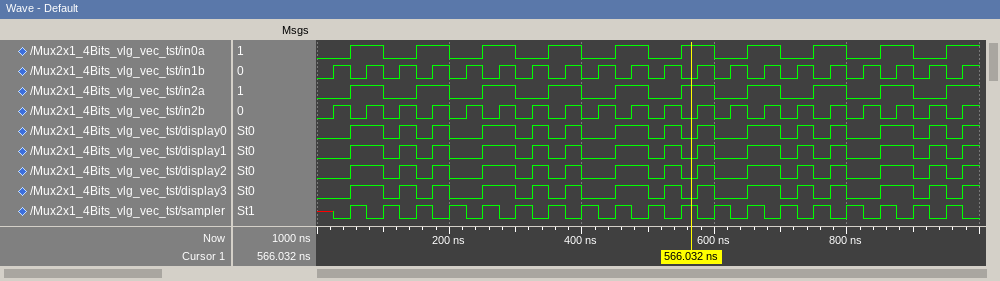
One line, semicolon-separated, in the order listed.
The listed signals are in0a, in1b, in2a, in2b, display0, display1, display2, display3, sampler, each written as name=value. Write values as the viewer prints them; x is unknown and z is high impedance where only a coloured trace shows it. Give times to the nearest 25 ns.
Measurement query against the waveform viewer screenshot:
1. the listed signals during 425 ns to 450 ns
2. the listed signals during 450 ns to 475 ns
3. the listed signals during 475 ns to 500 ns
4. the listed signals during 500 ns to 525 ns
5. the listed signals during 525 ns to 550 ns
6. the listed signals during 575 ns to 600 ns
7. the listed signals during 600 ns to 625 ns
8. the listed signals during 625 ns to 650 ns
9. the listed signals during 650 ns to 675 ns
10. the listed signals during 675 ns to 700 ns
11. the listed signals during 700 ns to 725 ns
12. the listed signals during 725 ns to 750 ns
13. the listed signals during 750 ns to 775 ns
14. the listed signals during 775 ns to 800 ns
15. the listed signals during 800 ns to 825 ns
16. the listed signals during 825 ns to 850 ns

in0a=0, in1b=1, in2a=0, in2b=1, display0=0, display1=0, display2=0, display3=0, sampler=0; in0a=1, in1b=0, in2a=1, in2b=0, display0=1, display1=1, display2=1, display3=1, sampler=1; in0a=1, in1b=1, in2a=1, in2b=1, display0=1, display1=1, display2=1, display3=1, sampler=0; in0a=0, in1b=0, in2a=0, in2b=0, display0=0, display1=0, display2=0, display3=0, sampler=1; in0a=0, in1b=1, in2a=0, in2b=1, display0=1, display1=1, display2=1, display3=1, sampler=0; in0a=1, in1b=1, in2a=1, in2b=1, display0=1, display1=1, display2=1, display3=1, sampler=0; in0a=0, in1b=0, in2a=0, in2b=0, display0=0, display1=0, display2=0, display3=0, sampler=1; in0a=0, in1b=1, in2a=0, in2b=1, display0=0, display1=0, display2=0, display3=0, sampler=0; in0a=1, in1b=0, in2a=1, in2b=0, display0=1, display1=1, display2=1, display3=1, sampler=1; in0a=1, in1b=1, in2a=1, in2b=1, display0=1, display1=1, display2=1, display3=1, sampler=0; in0a=0, in1b=0, in2a=0, in2b=0, display0=0, display1=0, display2=0, display3=0, sampler=1; in0a=0, in1b=1, in2a=0, in2b=1, display0=1, display1=1, display2=1, display3=1, sampler=0; in0a=1, in1b=0, in2a=1, in2b=0, display0=0, display1=0, display2=0, display3=0, sampler=1; in0a=1, in1b=1, in2a=1, in2b=1, display0=1, display1=1, display2=1, display3=1, sampler=0; in0a=0, in1b=0, in2a=0, in2b=0, display0=0, display1=0, display2=0, display3=0, sampler=1; in0a=0, in1b=1, in2a=0, in2b=1, display0=0, display1=0, display2=0, display3=0, sampler=0
